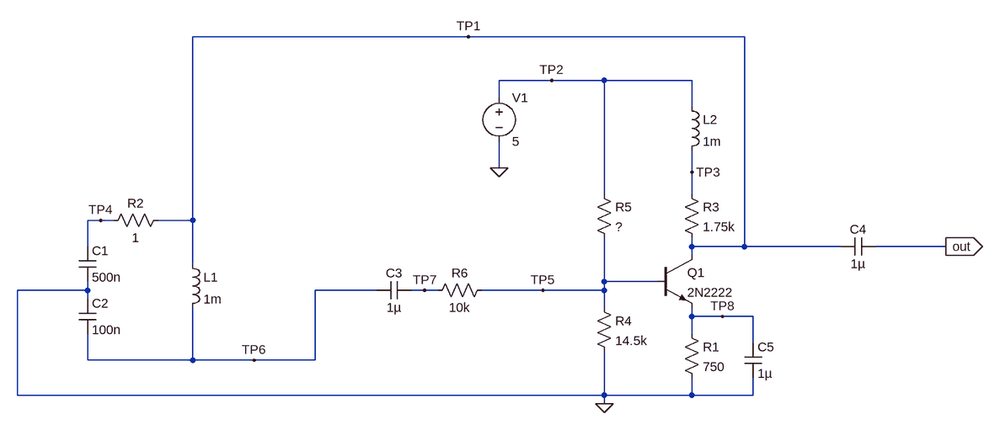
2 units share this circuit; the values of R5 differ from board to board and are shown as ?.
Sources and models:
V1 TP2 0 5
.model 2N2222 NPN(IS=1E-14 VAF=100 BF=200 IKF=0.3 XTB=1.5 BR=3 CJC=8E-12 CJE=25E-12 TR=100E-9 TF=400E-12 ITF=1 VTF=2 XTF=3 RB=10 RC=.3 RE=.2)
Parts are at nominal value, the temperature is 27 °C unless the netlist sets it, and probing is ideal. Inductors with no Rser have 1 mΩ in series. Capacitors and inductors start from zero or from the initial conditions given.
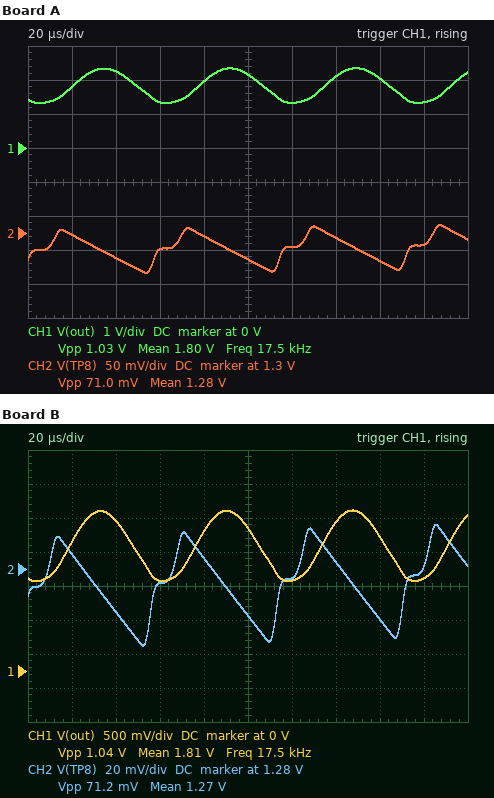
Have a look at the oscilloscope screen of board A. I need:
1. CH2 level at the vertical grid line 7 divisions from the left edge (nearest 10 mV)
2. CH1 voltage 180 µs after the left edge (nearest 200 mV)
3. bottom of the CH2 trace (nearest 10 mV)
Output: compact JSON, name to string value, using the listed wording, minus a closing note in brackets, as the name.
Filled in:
{"CH2 level at the vertical grid line 7 divisions from the left edge": "1.29 V", "CH1 voltage 180 µs after the left edge": "1.4 V", "bottom of the CH2 trace": "1.24 V"}
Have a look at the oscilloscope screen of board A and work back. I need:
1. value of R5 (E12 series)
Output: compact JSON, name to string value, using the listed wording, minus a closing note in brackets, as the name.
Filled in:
{"value of R5": "82 kΩ"}
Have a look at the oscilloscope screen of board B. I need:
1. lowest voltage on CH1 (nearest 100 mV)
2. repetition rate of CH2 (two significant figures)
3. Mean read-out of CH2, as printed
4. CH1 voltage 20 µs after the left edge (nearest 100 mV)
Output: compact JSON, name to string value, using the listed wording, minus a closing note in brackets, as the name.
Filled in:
{"lowest voltage on CH1": "1.3 V", "repetition rate of CH2": "18 kHz", "Mean read-out of CH2, as printed": "1.27 V", "CH1 voltage 20 µs after the left edge": "1.9 V"}
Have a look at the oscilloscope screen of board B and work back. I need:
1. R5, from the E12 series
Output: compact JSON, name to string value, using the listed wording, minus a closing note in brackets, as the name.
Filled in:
{"R5, from the E12 series": "100 kΩ"}
